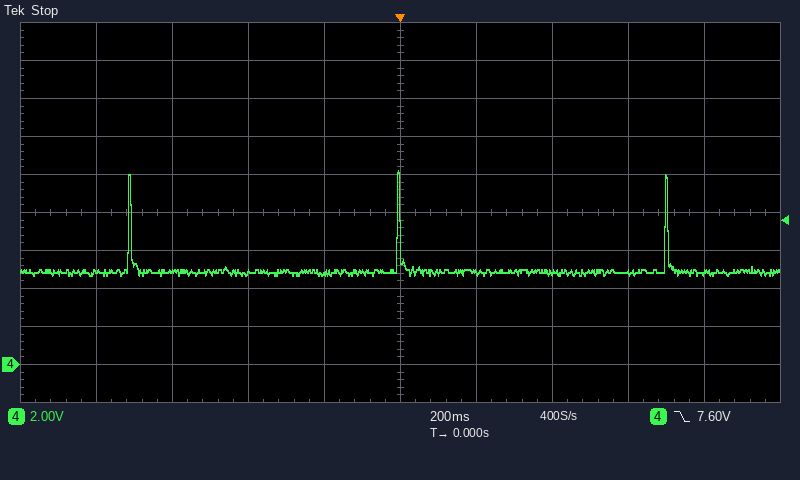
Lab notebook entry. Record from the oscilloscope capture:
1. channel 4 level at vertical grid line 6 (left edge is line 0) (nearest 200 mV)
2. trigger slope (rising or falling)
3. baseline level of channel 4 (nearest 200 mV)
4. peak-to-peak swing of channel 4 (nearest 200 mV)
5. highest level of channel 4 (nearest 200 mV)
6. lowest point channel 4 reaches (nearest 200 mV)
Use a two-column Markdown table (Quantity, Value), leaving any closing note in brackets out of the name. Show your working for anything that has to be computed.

| Quantity | Value |
|---|---|
| channel 4 level at vertical grid line 6 (left edge is line 0) | 4.8 V |
| trigger slope | falling |
| baseline level of channel 4 | 4.8 V |
| peak-to-peak swing of channel 4 | 10.2 V − (4.6 V) = 5.6 V |
| highest level of channel 4 | 10.2 V |
| lowest point channel 4 reaches | 4.6 V |
